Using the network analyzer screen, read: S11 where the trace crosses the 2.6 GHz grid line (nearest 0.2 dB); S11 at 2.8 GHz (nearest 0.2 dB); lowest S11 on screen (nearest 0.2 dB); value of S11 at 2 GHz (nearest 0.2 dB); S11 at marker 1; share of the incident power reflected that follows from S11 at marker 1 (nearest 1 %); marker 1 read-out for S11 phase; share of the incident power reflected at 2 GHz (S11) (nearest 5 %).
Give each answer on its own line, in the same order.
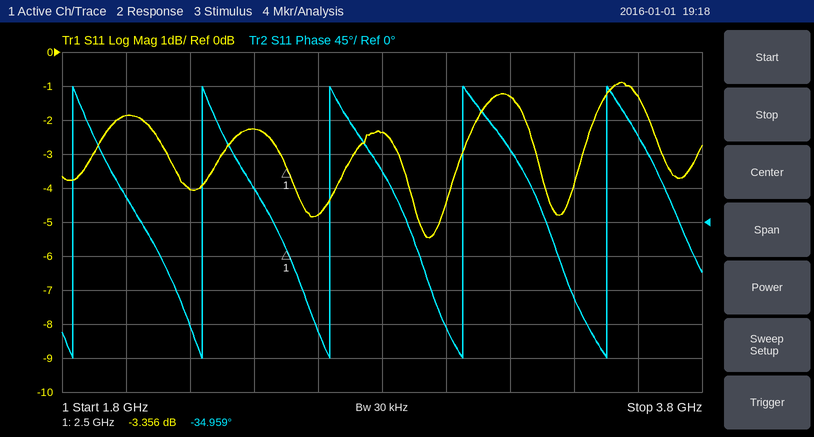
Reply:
-4.8 dB
-2.4 dB
-5.4 dB
-1.8 dB
-3.356 dB
46 %
-34.959°
65 %
